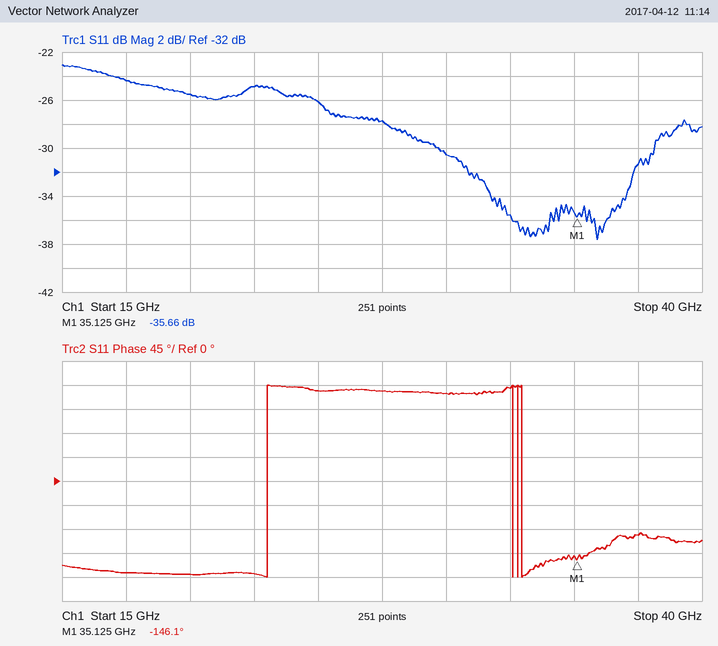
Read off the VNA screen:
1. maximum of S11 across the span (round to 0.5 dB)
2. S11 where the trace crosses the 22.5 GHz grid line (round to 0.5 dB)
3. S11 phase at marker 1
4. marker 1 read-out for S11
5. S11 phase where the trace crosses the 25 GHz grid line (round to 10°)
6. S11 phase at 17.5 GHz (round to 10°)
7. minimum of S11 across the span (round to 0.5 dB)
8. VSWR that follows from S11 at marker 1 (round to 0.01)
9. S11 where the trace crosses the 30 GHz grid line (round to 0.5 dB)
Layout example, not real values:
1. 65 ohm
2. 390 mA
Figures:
1. -23.0 dB
2. -25.0 dB
3. -146.1°
4. -35.66 dB
5. 170°
6. -170°
7. -37.5 dB
8. 1.03
9. -30.5 dB
